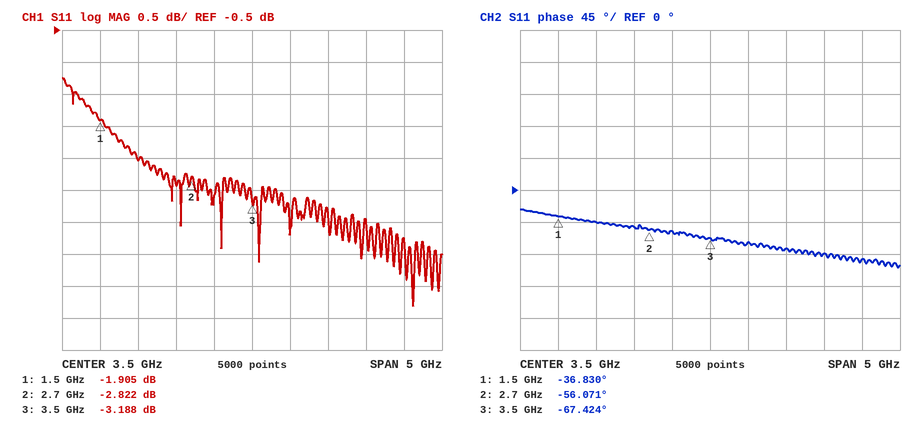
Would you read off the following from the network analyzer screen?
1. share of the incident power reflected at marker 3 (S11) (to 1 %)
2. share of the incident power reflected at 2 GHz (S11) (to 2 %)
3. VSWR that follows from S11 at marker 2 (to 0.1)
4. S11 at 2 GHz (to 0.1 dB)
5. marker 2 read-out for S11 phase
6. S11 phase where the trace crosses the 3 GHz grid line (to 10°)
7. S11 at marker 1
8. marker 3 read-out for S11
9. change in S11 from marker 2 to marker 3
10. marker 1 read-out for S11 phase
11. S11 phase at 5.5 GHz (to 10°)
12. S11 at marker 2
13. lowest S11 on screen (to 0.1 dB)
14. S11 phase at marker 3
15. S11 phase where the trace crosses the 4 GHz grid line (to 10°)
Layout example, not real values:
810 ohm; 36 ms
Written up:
48 %; 56 %; 6.2; -2.5 dB; -56.071°; -60°; -1.905 dB; -3.188 dB; -0.366 dB; -36.830°; -100°; -2.822 dB; -4.8 dB; -67.424°; -70°
